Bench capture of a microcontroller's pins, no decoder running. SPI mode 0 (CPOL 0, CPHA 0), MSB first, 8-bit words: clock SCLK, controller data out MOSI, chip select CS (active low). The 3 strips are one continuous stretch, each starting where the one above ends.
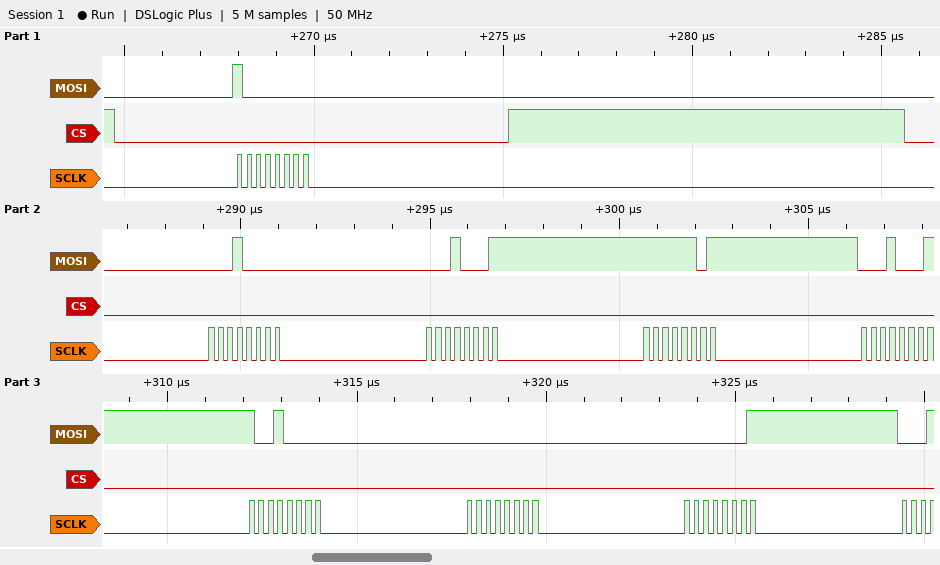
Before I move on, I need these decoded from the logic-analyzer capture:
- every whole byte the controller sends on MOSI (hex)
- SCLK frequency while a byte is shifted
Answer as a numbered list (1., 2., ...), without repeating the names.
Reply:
1. 0x80 0x10 0x11 0xFD 0x11 0x90 0x00 0x01
2. 4 MHz
